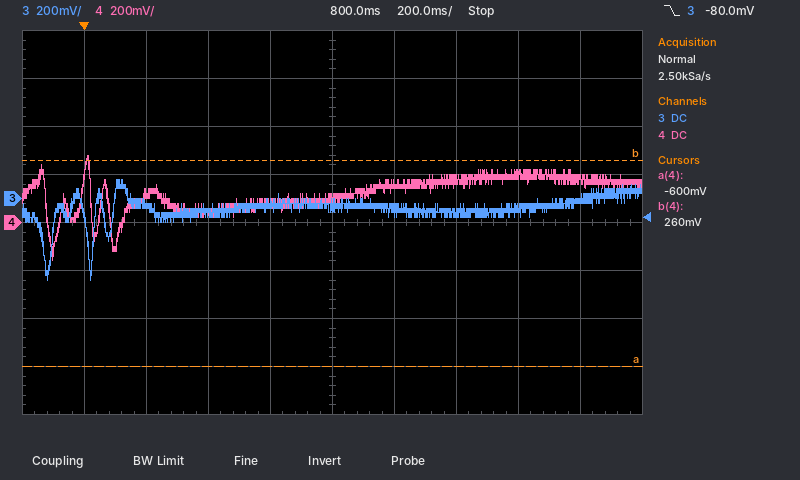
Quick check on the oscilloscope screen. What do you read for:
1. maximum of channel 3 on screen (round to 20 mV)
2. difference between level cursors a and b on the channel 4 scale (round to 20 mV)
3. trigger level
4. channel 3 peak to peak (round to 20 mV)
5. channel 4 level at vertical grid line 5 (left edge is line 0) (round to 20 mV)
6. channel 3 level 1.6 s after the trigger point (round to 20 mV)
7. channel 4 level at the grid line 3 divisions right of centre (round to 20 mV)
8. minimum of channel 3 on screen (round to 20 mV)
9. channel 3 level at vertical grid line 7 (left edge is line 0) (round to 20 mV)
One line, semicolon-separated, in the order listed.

80 mV; 860 mV; -80.0 mV; 420 mV; 100 mV; 0 mV; 200 mV; -340 mV; -60 mV
